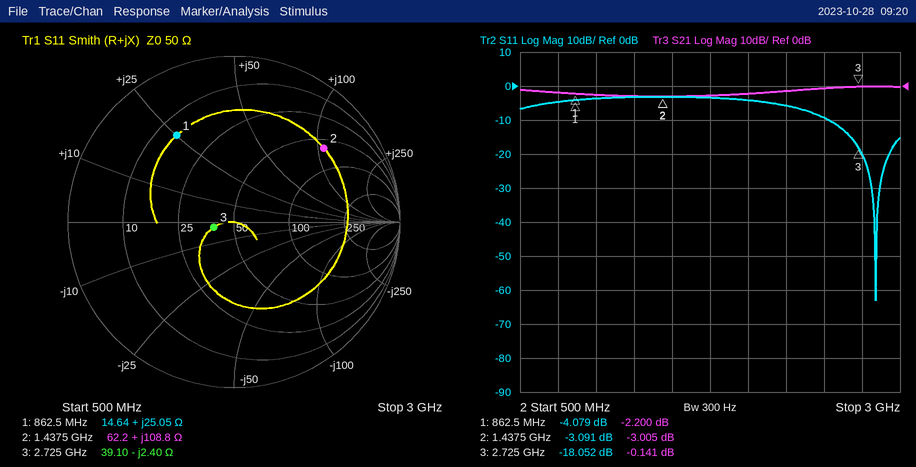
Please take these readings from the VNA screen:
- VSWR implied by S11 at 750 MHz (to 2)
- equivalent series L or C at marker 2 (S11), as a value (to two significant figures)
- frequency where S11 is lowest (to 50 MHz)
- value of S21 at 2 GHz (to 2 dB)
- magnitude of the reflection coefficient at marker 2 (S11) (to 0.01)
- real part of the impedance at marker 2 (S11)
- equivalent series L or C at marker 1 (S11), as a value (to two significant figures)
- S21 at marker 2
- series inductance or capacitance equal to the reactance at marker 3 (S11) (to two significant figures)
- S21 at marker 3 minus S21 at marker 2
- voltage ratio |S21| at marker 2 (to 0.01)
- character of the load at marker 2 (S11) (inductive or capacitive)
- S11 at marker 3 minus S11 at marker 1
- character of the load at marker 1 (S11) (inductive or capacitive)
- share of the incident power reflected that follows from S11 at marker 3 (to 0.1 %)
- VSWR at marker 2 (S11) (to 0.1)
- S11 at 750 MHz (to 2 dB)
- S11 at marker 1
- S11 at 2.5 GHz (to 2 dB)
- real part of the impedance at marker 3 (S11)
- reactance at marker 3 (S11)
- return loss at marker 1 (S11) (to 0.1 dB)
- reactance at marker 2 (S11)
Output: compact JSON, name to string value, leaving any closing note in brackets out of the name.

{"VSWR implied by S11 at 750 MHz": "4", "equivalent series L or C at marker 2 (S11), as a value": "12 nH", "frequency where S11 is lowest": "2.85 GHz", "value of S21 at 2 GHz": "-2 dB", "magnitude of the reflection coefficient at marker 2 (S11)": "0.70", "real part of the impedance at marker 2": "62.2 Ω", "equivalent series L or C at marker 1 (S11), as a value": "4.6 nH", "S21 at marker 2": "-3.005 dB", "series inductance or capacitance equal to the reactance at marker 3 (S11)": "24 pF", "S21 at marker 3 minus S21 at marker 2": "2.864 dB", "voltage ratio |S21| at marker 2": "0.71", "character of the load at marker 2 (S11)": "inductive", "S11 at marker 3 minus S11 at marker 1": "-13.973 dB", "character of the load at marker 1 (S11)": "inductive", "share of the incident power reflected that follows from S11 at marker 3": "1.6 %", "VSWR at marker 2 (S11)": "5.7", "S11 at 750 MHz": "-4 dB", "S11 at marker 1": "-4.079 dB", "S11 at 2.5 GHz": "-10 dB", "real part of the impedance at marker 3": "39.10 Ω", "reactance at marker 3": "-2.40 Ω", "return loss at marker 1 (S11)": "4.1 dB", "reactance at marker 2": "+108.8 Ω"}
